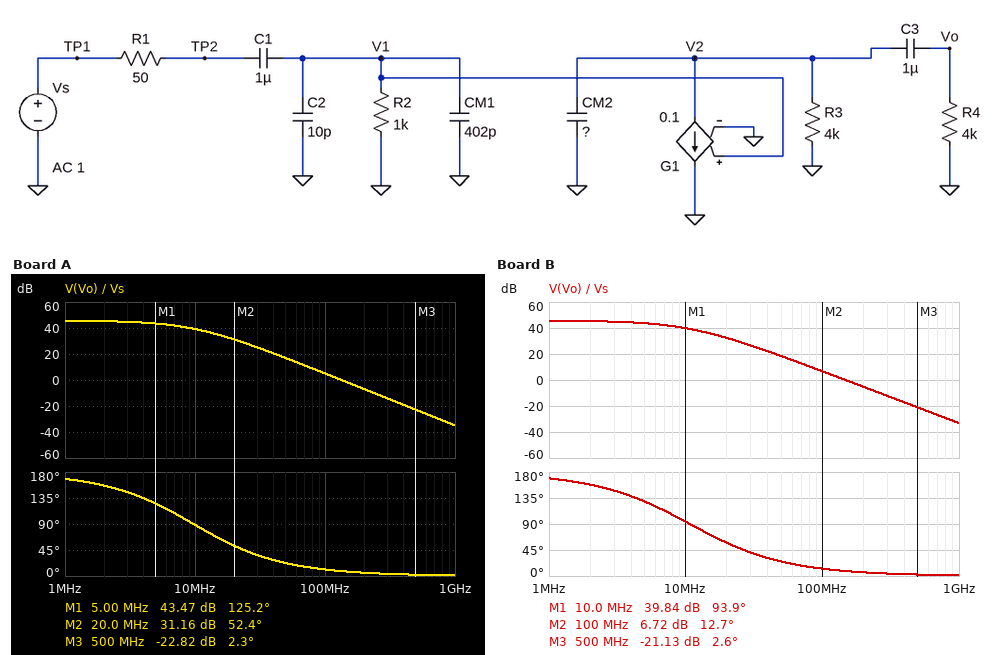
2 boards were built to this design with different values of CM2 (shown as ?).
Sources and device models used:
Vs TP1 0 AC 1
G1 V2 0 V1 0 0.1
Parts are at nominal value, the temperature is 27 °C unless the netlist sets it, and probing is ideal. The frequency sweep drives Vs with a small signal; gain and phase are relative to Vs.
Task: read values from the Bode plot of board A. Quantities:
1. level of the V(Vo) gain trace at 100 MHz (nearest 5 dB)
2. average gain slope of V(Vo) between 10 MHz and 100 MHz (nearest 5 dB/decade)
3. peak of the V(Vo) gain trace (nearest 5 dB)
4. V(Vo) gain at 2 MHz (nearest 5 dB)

5 dB
-35 dB/decade
45 dB
45 dB
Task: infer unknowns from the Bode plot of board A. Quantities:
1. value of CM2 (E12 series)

6.8 pF
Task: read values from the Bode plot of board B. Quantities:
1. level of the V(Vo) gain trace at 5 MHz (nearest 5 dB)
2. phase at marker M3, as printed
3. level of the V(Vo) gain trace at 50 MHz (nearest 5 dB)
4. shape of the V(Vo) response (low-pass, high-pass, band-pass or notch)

45 dB
2.6 deg
20 dB
low-pass
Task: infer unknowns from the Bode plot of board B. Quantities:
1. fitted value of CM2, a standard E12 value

5.6 pF
